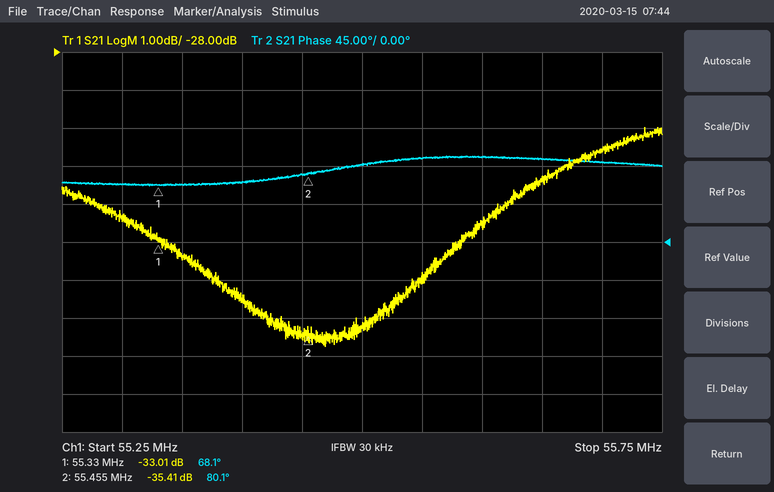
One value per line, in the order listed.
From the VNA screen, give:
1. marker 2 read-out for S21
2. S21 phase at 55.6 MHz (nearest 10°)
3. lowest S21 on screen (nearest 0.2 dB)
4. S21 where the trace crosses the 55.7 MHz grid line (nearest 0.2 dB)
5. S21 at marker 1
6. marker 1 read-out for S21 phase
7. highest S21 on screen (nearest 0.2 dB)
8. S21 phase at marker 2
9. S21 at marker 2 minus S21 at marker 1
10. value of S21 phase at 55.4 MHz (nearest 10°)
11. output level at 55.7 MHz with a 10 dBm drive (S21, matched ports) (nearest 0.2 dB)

-35.41 dB
100°
-35.8 dB
-30.6 dB
-33.01 dB
68.1°
-30.0 dB
80.1°
-2.40 dB
70°
-20.6 dBm
